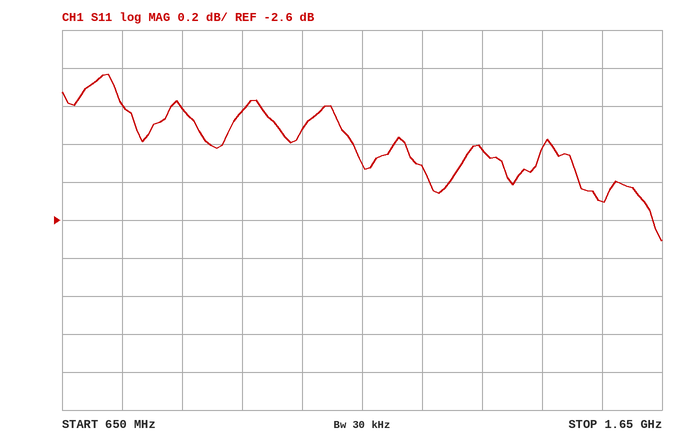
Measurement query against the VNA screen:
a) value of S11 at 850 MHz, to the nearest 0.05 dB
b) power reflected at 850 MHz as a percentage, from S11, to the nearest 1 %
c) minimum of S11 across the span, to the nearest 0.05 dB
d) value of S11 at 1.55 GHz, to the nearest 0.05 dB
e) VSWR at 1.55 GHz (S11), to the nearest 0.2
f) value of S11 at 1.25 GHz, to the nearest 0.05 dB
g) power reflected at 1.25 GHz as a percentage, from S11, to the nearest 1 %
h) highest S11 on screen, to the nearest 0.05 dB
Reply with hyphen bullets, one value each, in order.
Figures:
- -2.00 dB
- 63 %
- -2.70 dB
- -2.50 dB
- 7.0
- -2.30 dB
- 59 %
- -1.85 dB
